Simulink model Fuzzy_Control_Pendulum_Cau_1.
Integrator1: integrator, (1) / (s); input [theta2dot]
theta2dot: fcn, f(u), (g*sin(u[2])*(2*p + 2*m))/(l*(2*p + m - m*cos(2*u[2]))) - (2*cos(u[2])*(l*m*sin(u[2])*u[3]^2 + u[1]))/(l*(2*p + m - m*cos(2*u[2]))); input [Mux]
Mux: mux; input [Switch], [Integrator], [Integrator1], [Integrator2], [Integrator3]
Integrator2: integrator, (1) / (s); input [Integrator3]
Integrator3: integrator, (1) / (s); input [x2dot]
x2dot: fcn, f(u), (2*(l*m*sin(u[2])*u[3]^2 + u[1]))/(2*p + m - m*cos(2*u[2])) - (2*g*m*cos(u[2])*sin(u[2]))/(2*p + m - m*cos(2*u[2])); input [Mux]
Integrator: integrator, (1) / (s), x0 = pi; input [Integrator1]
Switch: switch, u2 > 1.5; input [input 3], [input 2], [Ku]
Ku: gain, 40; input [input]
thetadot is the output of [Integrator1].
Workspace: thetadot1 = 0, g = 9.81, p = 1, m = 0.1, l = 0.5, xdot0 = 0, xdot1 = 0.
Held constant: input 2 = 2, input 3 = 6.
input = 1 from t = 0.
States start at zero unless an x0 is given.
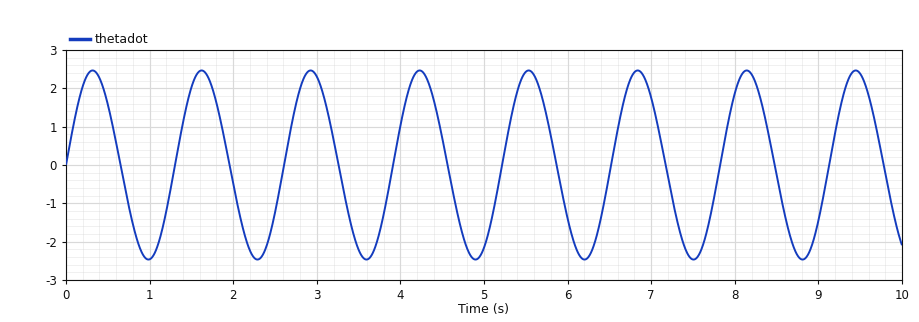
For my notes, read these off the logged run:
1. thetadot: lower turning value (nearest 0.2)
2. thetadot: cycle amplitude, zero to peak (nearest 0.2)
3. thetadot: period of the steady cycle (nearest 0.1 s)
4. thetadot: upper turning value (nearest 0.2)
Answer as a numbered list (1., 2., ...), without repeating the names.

1. -2.4
2. 2.4
3. 1.3 s
4. 2.4
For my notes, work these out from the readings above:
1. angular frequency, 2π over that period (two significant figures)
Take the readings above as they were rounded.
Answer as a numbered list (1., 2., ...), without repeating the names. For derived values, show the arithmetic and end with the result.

1. 2π / 1.3 = 4.8 rad/s
